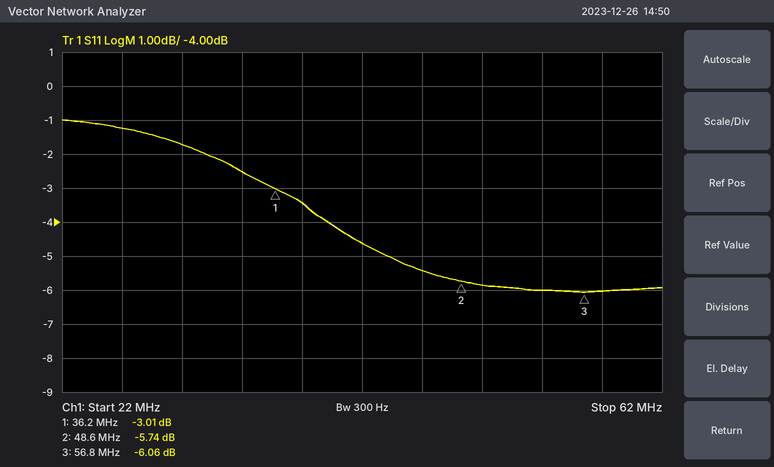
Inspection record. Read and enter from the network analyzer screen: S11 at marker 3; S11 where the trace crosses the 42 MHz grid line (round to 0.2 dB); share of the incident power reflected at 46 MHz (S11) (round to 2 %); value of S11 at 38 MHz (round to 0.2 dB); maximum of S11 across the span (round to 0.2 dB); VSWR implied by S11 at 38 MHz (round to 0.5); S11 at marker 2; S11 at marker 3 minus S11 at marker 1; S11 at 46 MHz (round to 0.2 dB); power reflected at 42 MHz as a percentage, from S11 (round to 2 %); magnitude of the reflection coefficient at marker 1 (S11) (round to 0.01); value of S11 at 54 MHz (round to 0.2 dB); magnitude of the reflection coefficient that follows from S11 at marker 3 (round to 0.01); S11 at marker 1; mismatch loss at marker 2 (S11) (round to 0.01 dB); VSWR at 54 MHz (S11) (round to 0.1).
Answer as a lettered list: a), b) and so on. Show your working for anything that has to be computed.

a) -6.06 dB
b) -4.6 dB
c) 10^(-5.4/10) ≈ 28.8 %, so 28 % to the nearest 2 %
d) -3.4 dB
e) -1.0 dB
f) |Γ| = 10^(-3.4/20) = 0.6761; VSWR = (1 + 0.6761)/(1 − 0.6761) ≈ 5.17, so 5.0 to the nearest 0.5
g) -5.74 dB
h) -6.06 − (-3.01) = -3.05 dB
i) -5.4 dB
j) 10^(-4.6/10) ≈ 34.7 %, so 34 % to the nearest 2 %
k) 10^(-3.01/20) ≈ 0.71
l) -6.0 dB
m) 10^(-6.06/20) ≈ 0.50
n) -3.01 dB
o) −10 log10(1 − 10^(-5.74/10)) ≈ 1.35 dB
p) |Γ| = 10^(-6/20) = 0.5012; VSWR = (1 + 0.5012)/(1 − 0.5012) ≈ 3.0
